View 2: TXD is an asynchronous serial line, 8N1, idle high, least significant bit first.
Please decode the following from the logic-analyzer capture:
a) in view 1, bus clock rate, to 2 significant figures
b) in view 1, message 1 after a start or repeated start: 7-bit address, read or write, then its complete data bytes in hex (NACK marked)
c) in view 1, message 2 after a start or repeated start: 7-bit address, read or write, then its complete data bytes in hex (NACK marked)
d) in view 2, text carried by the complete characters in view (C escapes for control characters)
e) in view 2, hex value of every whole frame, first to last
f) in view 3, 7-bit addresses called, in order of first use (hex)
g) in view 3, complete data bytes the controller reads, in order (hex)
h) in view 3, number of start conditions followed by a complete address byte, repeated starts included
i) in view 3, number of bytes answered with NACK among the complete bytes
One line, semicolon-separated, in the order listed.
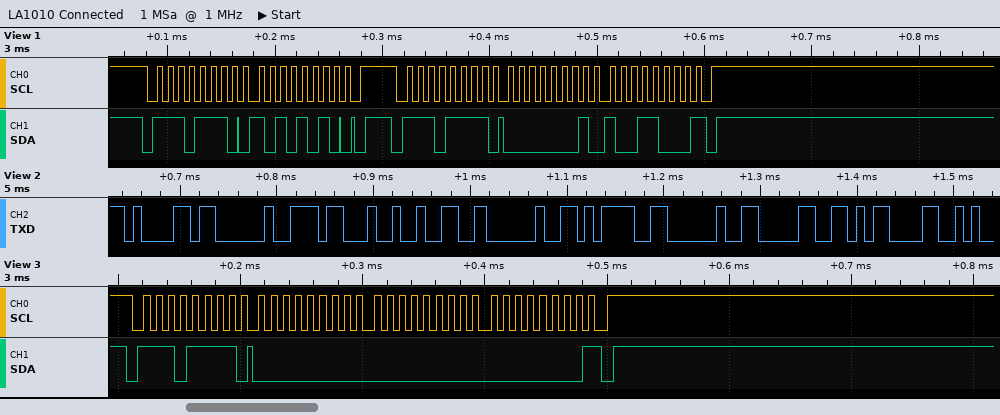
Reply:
100 kHz; 0x77 write: AA; 0x77 read: 01 98 NACK; "a #2 = 0\r"; 61 20 23 32 20 3D 20 30 0D; 0x77; 00 00 00; 1; 1
